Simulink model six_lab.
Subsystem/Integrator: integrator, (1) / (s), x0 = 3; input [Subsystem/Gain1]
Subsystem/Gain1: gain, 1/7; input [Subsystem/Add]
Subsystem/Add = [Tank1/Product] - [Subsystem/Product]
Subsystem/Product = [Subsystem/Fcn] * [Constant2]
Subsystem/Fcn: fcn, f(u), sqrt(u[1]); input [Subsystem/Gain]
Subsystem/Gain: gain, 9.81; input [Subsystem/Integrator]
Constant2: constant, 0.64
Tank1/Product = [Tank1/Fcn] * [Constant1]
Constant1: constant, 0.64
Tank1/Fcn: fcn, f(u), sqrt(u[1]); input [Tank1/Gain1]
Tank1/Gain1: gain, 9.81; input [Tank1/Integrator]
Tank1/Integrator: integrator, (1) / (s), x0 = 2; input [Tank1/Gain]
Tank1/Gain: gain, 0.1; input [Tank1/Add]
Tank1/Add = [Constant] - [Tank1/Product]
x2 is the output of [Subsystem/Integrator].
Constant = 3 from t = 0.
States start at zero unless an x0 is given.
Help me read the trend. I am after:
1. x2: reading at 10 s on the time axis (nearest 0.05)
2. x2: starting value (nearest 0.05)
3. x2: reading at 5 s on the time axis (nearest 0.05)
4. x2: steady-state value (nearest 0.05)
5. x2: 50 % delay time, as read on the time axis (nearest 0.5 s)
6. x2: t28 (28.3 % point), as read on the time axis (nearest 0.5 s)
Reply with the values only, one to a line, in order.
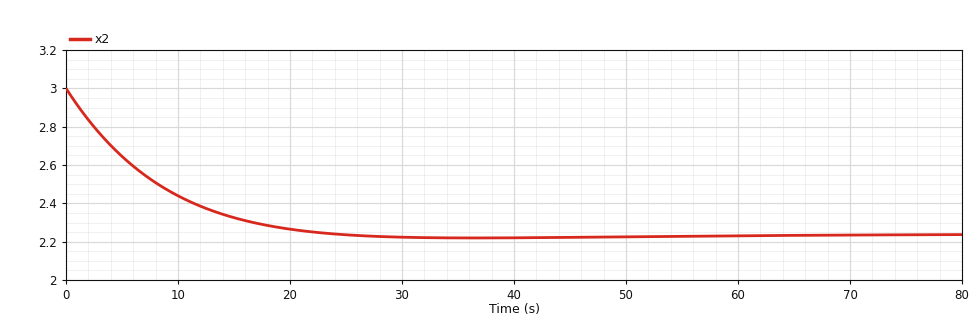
2.45
3.00
2.65
2.25
5.5 s
2.5 s
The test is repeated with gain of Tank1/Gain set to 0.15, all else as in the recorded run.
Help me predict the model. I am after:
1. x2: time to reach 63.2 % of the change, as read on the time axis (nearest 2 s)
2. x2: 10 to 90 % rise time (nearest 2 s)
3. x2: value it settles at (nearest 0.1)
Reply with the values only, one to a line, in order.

8 s
16 s
2.2
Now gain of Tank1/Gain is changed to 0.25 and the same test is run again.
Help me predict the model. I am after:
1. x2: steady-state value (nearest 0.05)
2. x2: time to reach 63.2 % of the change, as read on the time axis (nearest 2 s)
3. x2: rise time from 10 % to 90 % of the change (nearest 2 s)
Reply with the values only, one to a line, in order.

2.25
8 s
20 s
